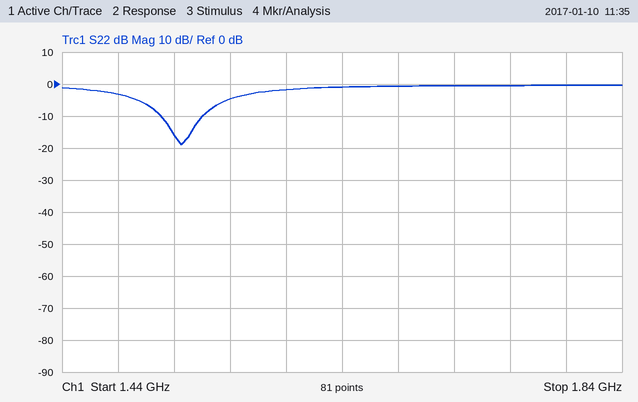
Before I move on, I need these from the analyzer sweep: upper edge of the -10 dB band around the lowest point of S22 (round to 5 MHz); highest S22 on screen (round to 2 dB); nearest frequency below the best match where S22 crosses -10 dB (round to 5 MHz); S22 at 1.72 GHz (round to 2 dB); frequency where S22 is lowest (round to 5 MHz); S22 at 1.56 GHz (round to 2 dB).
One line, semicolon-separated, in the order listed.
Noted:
1.540 GHz; 0 dB; 1.510 GHz; 0 dB; 1.525 GHz; -4 dB
